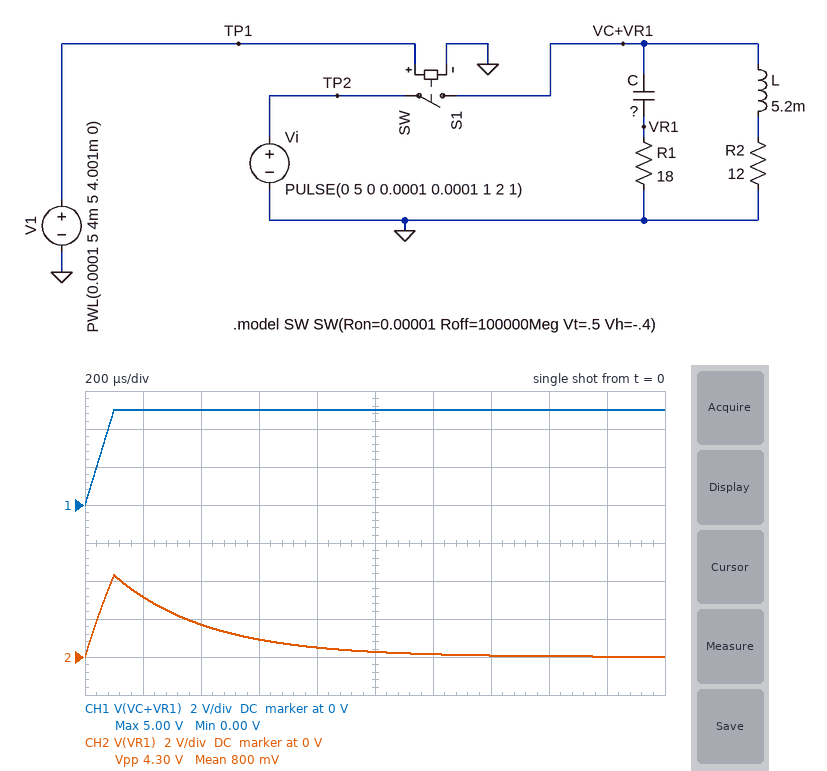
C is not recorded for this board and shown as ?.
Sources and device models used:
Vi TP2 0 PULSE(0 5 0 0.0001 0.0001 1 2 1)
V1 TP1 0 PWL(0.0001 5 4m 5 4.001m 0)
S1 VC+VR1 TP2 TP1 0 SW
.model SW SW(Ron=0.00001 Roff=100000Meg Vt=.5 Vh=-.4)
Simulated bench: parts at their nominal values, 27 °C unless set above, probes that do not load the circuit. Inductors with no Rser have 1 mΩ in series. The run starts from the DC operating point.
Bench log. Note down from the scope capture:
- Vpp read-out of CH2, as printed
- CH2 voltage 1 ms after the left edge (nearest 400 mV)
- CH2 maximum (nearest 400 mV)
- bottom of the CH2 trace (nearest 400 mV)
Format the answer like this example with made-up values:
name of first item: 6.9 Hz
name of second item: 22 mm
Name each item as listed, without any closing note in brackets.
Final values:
Vpp read-out of CH2, as printed: 4.30 V
CH2 voltage 1 ms after the left edge: 400 mV
CH2 maximum: 4.4 V
bottom of the CH2 trace: 0 V
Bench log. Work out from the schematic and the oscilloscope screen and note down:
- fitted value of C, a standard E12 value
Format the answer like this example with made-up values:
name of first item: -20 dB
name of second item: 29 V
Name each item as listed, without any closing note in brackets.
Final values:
fitted value of C, a standard E12 value: 18 µF
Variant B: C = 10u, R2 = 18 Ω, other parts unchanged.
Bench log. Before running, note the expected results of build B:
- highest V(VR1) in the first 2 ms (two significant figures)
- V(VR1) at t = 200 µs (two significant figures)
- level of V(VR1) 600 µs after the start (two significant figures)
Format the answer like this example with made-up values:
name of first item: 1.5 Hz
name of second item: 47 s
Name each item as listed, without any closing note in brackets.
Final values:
highest V(VR1) in the first 2 ms: 3.8 V
V(VR1) at t = 200 µs: 2.2 V
level of V(VR1) 600 µs after the start: 240 mV
